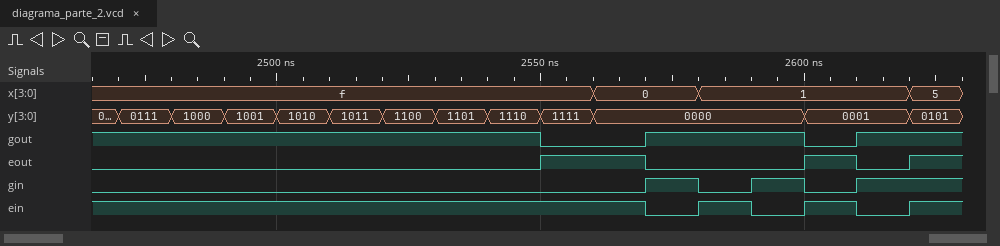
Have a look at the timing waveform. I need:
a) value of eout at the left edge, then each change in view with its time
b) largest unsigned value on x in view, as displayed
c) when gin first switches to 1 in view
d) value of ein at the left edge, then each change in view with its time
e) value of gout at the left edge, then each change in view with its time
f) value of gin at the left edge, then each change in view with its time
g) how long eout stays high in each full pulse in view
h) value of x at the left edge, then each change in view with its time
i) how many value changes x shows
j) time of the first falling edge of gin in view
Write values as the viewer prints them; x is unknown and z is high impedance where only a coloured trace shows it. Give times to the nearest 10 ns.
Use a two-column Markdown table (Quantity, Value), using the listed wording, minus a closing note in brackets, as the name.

| Quantity | Value |
|---|---|
| value of eout at the left edge, then each change in view with its time | 0, 1 at 2550 ns, 0 at 2570 ns, 1 at 2600 ns, 0 at 2610 ns, 1 at 2620 ns |
| largest unsigned value on x in view, as displayed | f |
| when gin first switches to 1 in view | 2570 ns |
| value of ein at the left edge, then each change in view with its time | 1, 0 at 2570 ns, 1 at 2580 ns, 0 at 2590 ns, 1 at 2600 ns, 0 at 2610 ns, 1 at 2620 ns |
| value of gout at the left edge, then each change in view with its time | 1, 0 at 2550 ns, 1 at 2570 ns, 0 at 2600 ns, 1 at 2610 ns |
| value of gin at the left edge, then each change in view with its time | 0, 1 at 2570 ns, 0 at 2580 ns, 1 at 2590 ns, 0 at 2600 ns, 1 at 2610 ns |
| how long eout stays high in each full pulse in view | 20 ns, 10 ns |
| value of x at the left edge, then each change in view with its time | f, 0 at 2560 ns, 1 at 2580 ns, 5 at 2620 ns |
| how many value changes x shows | 3 |
| time of the first falling edge of gin in view | 2580 ns |
